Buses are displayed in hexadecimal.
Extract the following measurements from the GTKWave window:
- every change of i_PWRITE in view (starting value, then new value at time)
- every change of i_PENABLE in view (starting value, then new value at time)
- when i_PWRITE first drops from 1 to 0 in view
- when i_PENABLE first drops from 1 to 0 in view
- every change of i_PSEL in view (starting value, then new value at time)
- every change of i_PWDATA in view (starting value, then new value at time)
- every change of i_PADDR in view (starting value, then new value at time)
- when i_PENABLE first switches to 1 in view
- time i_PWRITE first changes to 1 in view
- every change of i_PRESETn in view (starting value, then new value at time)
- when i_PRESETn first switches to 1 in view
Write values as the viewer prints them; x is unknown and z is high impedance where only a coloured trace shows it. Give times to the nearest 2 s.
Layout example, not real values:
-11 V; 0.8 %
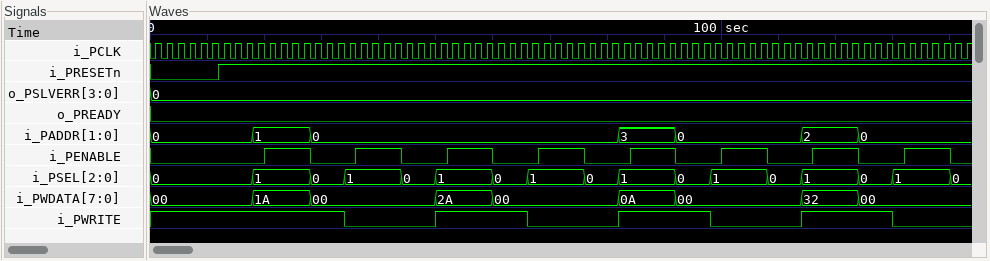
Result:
1, 0 at 34 s, 1 at 50 s, 0 at 66 s, 1 at 82 s, 0 at 98 s, 1 at 114 s, 0 at 130 s; 0, 1 at 20 s, 0 at 28 s, 1 at 36 s, 0 at 44 s, 1 at 52 s, 0 at 60 s, 1 at 68 s, 0 at 76 s, 1 at 84 s, 0 at 92 s, 1 at 100 s, 0 at 108 s, 1 at 116 s, 0 at 124 s, 1 at 132 s, 0 at 140 s; 34 s; 28 s; 0, 1 at 18 s, 0 at 28 s, 1 at 34 s, 0 at 44 s, 1 at 50 s, 0 at 60 s, 1 at 66 s, 0 at 76 s, 1 at 82 s, 0 at 92 s, 1 at 98 s, 0 at 108 s, 1 at 114 s, 0 at 124 s, 1 at 130 s, 0 at 140 s; 00, 1A at 18 s, 00 at 28 s, 2A at 50 s, 00 at 60 s, 0A at 82 s, 00 at 92 s, 32 at 114 s, 00 at 124 s; 0, 1 at 18 s, 0 at 28 s, 3 at 82 s, 0 at 92 s, 2 at 114 s, 0 at 124 s; 20 s; 50 s; 0, 1 at 12 s; 12 s
